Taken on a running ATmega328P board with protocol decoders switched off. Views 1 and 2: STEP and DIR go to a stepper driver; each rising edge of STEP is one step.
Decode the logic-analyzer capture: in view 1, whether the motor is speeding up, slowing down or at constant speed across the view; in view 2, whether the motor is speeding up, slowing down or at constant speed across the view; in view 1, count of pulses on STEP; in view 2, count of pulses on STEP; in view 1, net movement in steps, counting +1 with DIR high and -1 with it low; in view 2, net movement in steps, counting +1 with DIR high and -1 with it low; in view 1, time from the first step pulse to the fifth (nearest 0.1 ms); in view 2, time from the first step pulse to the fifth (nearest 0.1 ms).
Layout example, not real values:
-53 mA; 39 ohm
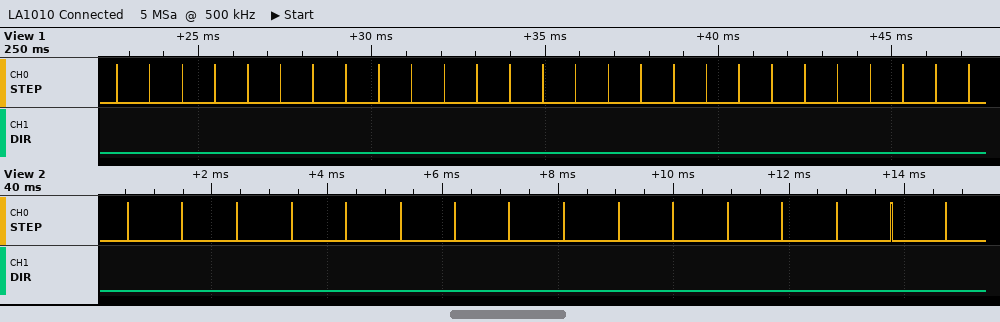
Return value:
constant speed; constant speed; 27; 16; -27; -16; 3.8 ms; 3.8 ms
